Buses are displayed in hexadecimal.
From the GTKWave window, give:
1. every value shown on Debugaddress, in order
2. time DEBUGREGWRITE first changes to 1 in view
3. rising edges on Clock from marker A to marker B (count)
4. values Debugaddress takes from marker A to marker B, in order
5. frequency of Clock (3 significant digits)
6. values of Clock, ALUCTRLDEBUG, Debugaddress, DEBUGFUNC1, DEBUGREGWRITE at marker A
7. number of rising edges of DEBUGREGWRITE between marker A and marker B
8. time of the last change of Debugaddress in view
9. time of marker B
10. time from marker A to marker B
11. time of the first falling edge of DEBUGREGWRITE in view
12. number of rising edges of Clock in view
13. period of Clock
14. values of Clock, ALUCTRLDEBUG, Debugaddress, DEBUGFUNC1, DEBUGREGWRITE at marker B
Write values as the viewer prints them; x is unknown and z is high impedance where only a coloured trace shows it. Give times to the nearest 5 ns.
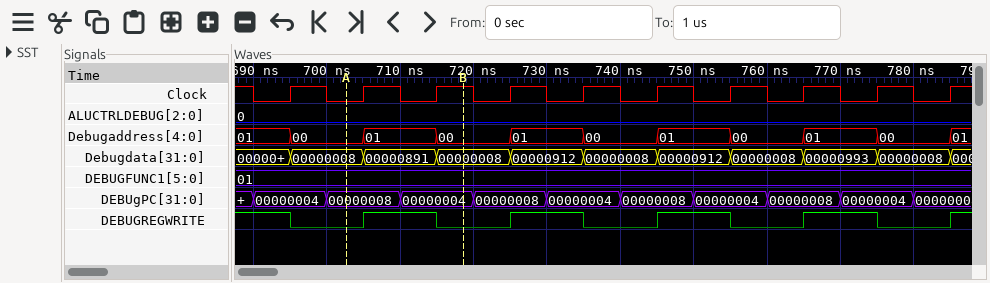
01, 00, 01, 00, 01, 00, 01, 00, 01, 00, 01
705 ns
2
00, 01, 00
100 MHz
Clock=0, ALUCTRLDEBUG=0, Debugaddress=00, DEBUGFUNC1=01, DEBUGREGWRITE=0
1
785 ns
720 ns
15 ns
695 ns
10
10 ns
Clock=1, ALUCTRLDEBUG=0, Debugaddress=00, DEBUGFUNC1=01, DEBUGREGWRITE=0
